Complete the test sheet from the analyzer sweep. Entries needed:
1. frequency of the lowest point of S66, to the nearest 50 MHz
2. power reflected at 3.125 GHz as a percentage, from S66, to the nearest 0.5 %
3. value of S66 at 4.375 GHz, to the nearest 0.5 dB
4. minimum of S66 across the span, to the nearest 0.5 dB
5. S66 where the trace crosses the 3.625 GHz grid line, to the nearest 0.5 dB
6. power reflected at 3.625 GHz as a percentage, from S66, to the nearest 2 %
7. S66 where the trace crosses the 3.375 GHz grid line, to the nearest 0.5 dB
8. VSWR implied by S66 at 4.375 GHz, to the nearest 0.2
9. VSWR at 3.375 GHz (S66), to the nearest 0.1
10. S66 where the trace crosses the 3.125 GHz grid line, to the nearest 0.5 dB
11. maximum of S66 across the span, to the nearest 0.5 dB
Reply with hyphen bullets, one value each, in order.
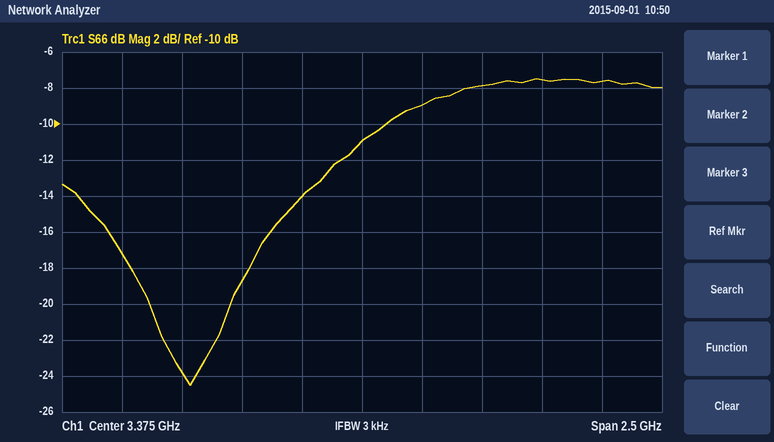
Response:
- 2.65 GHz
- 4.0 %
- -7.5 dB
- -24.5 dB
- -9.0 dB
- 12 %
- -11.0 dB
- 2.4
- 1.8
- -14.0 dB
- -7.5 dB
